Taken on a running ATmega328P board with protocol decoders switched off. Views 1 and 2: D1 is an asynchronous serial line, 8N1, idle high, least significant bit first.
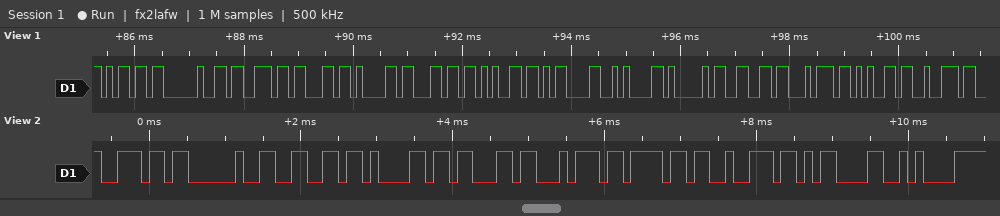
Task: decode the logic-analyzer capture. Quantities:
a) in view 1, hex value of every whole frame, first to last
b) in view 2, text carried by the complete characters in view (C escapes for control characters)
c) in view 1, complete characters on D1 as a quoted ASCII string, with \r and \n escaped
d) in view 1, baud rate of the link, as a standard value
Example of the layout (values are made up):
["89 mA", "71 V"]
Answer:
["6D 20 73 63 61 6C 65 0D 0A 41 66 74 65 72", "\"n factor\\r\\n\"", "\"m scale\\r\\nAfter\"", "9600 baud"]
